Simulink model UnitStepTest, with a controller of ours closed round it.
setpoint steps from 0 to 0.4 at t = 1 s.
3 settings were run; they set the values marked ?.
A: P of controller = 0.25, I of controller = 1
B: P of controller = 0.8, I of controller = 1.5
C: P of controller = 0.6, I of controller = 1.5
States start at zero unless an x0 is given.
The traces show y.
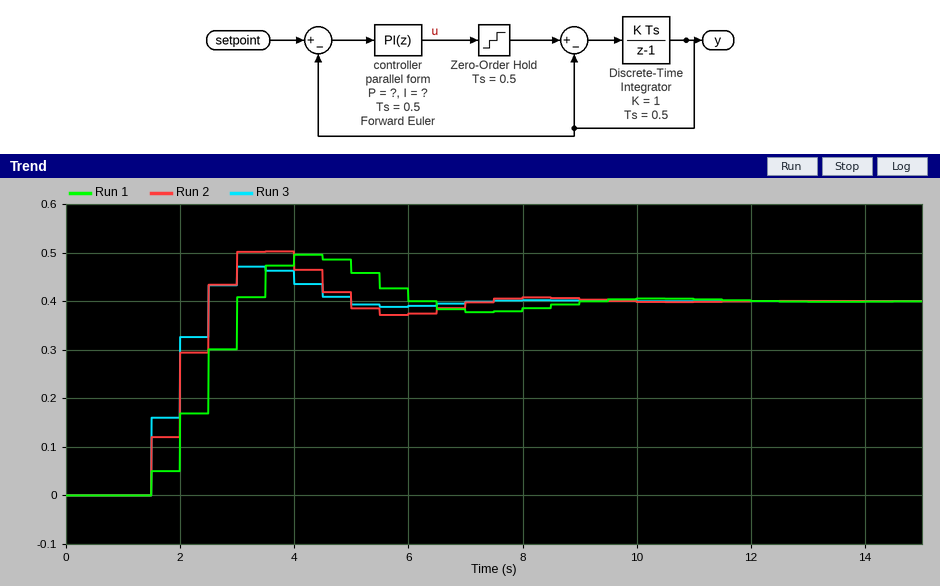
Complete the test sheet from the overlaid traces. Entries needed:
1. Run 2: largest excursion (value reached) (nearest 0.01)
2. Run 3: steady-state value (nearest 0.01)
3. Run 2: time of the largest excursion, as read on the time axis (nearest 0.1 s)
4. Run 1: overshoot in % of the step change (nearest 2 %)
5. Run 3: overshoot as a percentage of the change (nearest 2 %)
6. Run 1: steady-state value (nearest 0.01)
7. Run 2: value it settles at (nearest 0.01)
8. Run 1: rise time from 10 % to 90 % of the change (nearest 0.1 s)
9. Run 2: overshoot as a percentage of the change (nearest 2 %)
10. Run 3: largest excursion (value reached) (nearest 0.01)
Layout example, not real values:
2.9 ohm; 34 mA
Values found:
0.50; 0.40; 3.5 s; 24 %; 18 %; 0.40; 0.40; 1.5 s; 26 %; 0.47
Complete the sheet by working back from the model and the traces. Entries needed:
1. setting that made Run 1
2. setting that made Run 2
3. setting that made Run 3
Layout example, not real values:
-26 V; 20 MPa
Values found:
A; C; B
